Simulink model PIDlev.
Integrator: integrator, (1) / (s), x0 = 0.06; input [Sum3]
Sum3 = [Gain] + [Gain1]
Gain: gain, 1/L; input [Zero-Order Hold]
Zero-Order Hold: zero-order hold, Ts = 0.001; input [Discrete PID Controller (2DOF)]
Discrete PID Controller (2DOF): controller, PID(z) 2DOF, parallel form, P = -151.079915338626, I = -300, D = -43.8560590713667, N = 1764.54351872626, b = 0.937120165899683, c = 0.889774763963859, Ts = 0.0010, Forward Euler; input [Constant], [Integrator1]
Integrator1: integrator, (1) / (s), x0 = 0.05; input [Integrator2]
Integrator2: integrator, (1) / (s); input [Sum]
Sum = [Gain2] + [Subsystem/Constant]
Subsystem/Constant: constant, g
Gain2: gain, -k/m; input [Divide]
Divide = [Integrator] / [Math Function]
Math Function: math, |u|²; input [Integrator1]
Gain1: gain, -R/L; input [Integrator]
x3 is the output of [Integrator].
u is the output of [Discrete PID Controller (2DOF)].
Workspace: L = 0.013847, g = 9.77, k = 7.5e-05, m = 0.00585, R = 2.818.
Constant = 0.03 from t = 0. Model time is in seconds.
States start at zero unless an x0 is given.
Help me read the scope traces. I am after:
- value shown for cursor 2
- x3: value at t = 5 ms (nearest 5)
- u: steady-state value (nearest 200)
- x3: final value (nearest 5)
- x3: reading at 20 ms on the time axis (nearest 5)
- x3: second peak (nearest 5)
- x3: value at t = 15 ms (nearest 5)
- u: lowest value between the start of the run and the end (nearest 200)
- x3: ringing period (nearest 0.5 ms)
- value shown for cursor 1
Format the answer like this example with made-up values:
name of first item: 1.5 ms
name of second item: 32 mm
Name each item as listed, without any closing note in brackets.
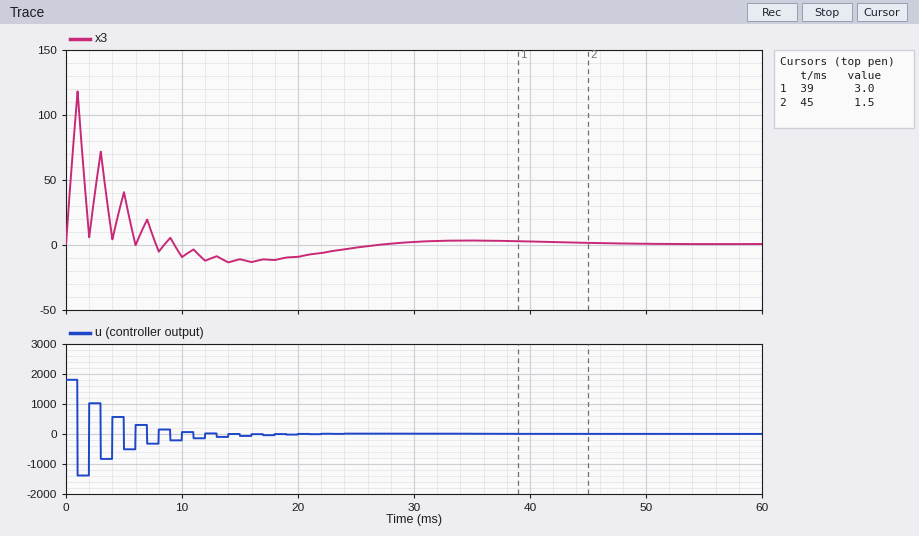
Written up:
value shown for cursor 2: 1.5
x3: value at t = 5 ms: 40
u: steady-state value: 0
x3: final value: 0
x3: reading at 20 ms on the time axis: -10
x3: second peak: 70
x3: value at t = 15 ms: -10
u: lowest value between the start of the run and the end: -1400
x3: ringing period: 2.0 ms
value shown for cursor 1: 3.0
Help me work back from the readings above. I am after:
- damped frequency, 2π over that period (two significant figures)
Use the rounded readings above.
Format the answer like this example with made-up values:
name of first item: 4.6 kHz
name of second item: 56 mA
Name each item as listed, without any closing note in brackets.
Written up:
damped frequency, 2π over that period: 3.1 rad/ms
